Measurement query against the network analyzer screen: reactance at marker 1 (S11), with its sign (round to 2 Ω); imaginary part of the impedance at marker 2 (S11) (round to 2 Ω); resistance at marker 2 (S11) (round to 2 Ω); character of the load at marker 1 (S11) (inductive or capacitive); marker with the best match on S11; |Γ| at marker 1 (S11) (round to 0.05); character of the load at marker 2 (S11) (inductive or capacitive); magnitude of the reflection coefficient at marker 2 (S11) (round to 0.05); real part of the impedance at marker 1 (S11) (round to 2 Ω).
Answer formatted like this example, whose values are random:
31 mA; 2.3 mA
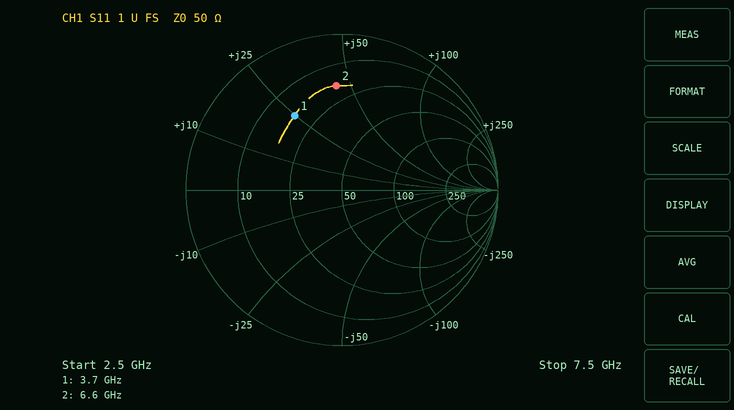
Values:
+24 Ω; +44 Ω; 18 Ω; inductive; marker 1; 0.55; inductive; 0.65; 18 Ω
